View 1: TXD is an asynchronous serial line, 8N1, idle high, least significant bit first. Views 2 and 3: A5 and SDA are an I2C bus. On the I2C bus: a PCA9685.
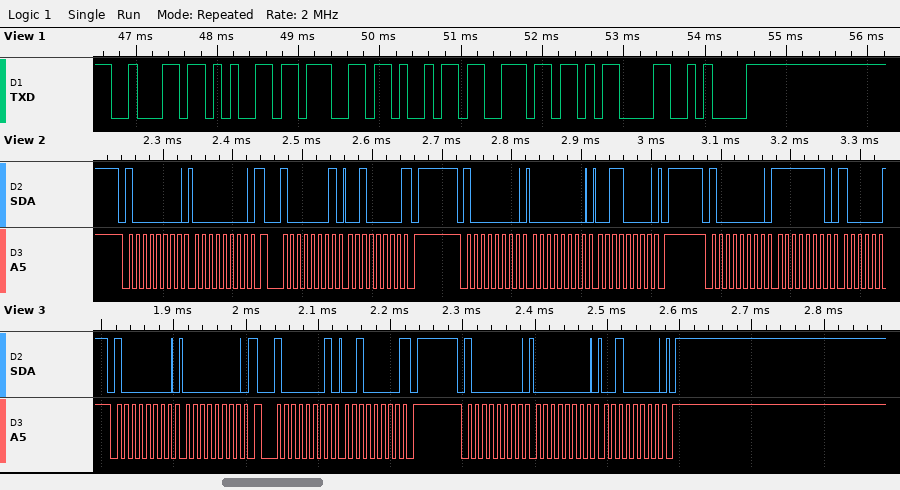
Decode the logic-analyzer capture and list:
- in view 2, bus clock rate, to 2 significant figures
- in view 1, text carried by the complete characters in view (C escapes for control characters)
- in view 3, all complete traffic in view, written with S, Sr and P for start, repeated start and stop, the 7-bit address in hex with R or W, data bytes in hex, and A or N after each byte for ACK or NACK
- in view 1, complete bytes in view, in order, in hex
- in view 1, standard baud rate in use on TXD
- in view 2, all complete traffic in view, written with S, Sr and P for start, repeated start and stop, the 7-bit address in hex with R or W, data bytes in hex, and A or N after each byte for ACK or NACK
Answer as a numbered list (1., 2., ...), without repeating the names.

1. 100 kHz
2. "begin\r\n"
3. S 40W A 00 A Sr 40R A 20 N P S 40W A 00 A 20 A P
4. 62 65 67 69 6E 0D 0A
5. 9600 baud
6. S 40W A 00 A Sr 40R A 20 N P S 40W A 00 A 30 A P S 40W A FE A
